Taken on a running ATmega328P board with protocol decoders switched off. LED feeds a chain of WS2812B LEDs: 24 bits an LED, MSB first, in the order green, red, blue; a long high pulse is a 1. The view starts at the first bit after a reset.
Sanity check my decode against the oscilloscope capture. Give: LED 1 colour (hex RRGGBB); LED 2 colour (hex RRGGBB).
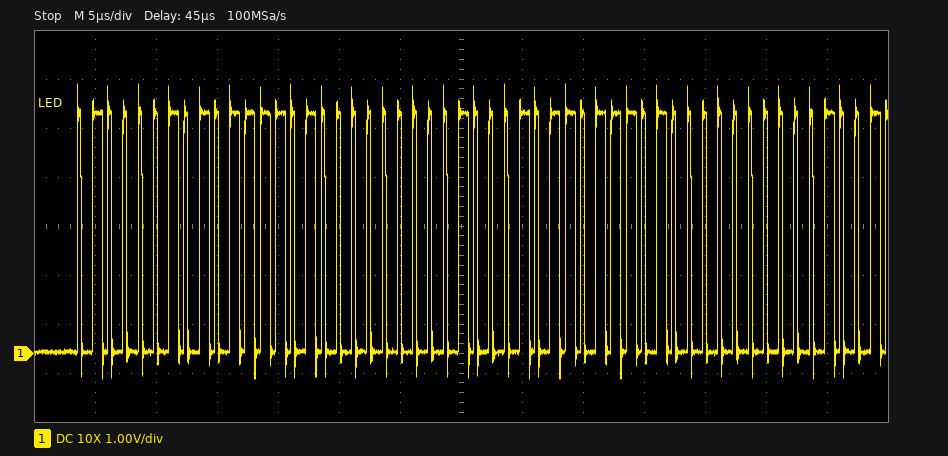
#BD4200
#BA4500
